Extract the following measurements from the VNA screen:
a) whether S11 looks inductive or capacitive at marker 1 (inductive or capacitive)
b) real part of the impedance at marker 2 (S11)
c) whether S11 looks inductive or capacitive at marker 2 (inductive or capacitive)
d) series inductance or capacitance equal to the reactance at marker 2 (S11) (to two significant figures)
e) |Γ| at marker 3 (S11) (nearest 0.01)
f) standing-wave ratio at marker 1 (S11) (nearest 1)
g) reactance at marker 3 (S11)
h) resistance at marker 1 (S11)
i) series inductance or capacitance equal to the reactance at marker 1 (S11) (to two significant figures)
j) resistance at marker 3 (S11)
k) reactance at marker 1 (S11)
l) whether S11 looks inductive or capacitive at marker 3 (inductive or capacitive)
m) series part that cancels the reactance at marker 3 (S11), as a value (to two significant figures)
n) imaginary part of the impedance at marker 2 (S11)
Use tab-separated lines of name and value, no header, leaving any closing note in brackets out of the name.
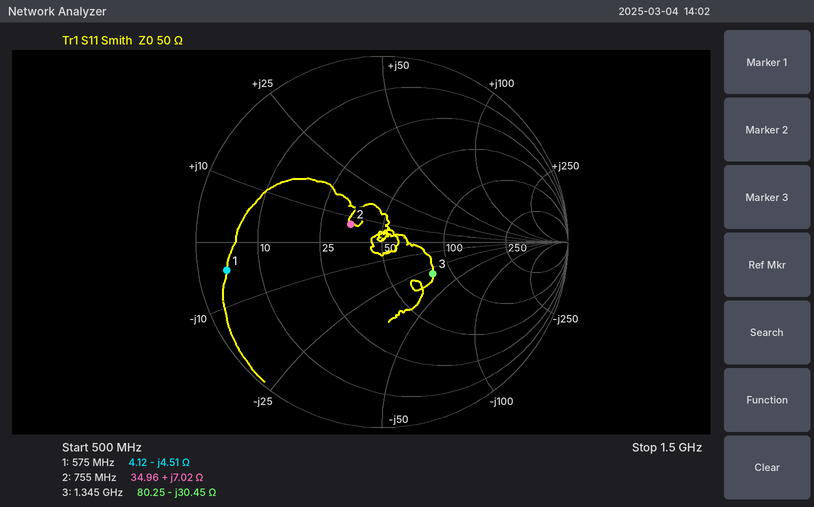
whether S11 looks inductive or capacitive at marker 1	capacitive
real part of the impedance at marker 2	34.96 Ω
whether S11 looks inductive or capacitive at marker 2	inductive
series inductance or capacitance equal to the reactance at marker 2 (S11)	1.5 nH
|Γ| at marker 3 (S11)	0.32
standing-wave ratio at marker 1 (S11)	12
reactance at marker 3	-30.45 Ω
resistance at marker 1	4.12 Ω
series inductance or capacitance equal to the reactance at marker 1 (S11)	61 pF
resistance at marker 3	80.25 Ω
reactance at marker 1	-4.51 Ω
whether S11 looks inductive or capacitive at marker 3	capacitive
series part that cancels the reactance at marker 3 (S11), as a value	3.6 nH
imaginary part of the impedance at marker 2	+7.02 Ω
